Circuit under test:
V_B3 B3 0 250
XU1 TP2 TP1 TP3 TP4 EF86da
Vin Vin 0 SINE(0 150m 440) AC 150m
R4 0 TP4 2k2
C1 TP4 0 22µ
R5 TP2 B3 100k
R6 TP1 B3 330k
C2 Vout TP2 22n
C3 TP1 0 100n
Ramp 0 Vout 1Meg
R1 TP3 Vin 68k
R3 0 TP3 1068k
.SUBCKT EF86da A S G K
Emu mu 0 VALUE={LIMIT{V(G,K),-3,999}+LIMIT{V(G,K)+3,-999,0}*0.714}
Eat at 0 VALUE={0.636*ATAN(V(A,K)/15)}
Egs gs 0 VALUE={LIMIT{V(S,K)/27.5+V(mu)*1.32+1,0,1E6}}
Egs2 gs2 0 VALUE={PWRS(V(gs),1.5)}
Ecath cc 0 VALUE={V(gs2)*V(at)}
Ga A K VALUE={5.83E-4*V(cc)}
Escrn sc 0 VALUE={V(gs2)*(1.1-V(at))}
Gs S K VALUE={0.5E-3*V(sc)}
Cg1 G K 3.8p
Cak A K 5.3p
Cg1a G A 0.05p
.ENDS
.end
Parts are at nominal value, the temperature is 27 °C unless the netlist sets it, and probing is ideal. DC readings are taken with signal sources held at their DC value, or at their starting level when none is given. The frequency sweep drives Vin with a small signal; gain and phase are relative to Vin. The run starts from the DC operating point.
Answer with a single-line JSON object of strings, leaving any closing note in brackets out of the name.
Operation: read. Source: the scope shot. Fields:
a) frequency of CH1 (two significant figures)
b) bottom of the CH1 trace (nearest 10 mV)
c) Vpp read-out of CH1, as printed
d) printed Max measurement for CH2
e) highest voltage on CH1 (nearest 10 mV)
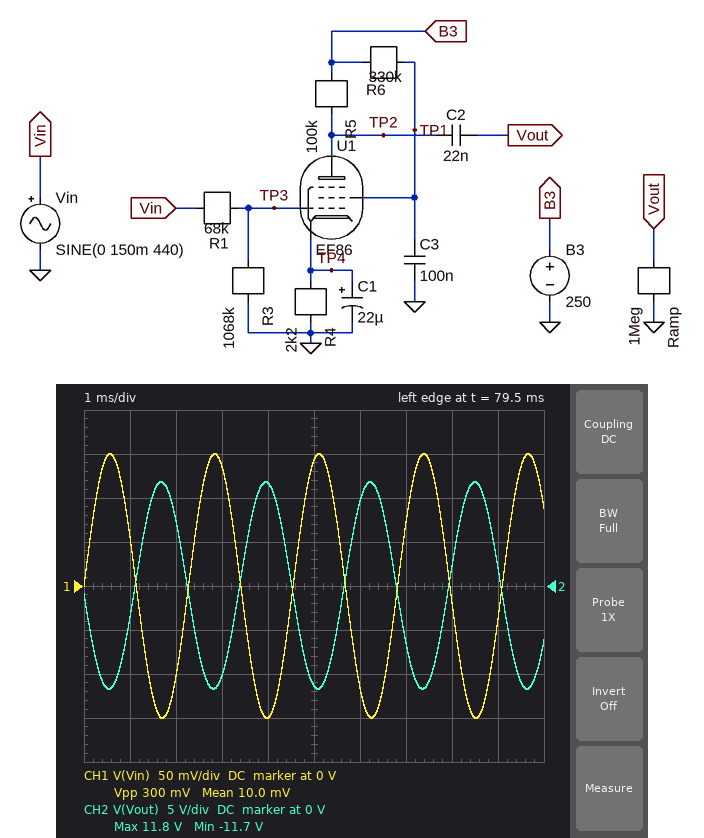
{"frequency of CH1": "440 Hz", "bottom of the CH1 trace": "-150 mV", "Vpp read-out of CH1, as printed": "300 mV", "printed Max measurement for CH2": "11.8 V", "highest voltage on CH1": "150 mV"}
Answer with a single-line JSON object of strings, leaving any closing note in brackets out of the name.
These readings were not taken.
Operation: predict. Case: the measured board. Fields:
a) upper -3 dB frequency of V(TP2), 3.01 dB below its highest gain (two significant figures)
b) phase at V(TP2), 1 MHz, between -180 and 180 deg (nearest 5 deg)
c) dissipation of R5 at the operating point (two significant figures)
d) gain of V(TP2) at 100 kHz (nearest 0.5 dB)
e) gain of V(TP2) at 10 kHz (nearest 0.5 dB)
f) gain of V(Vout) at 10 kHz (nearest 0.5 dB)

{"upper -3 dB frequency of V(TP2), 3.01 dB below its highest gain": "190 kHz", "phase at V(TP2), 1 MHz, between -180 and 180 deg": "60 deg", "dissipation of R5 at the operating point": "210 mW", "gain of V(TP2) at 100 kHz": "37.0 dB", "gain of V(TP2) at 10 kHz": "38.0 dB", "gain of V(Vout) at 10 kHz": "38.0 dB"}
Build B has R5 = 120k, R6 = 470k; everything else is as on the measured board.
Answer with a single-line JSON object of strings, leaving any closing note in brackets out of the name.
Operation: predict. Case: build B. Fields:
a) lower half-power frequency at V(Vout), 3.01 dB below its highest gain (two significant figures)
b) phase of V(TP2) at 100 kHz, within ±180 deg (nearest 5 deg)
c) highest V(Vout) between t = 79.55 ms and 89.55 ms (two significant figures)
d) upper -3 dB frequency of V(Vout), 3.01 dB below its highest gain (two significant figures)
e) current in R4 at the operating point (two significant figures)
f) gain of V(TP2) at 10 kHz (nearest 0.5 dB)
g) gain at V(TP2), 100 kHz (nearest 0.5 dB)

{"lower half-power frequency at V(Vout), 3.01 dB below its highest gain": "31 Hz", "phase of V(TP2) at 100 kHz, within ±180 deg": "145 deg", "highest V(Vout) between t = 79.55 ms and 89.55 ms": "13 V", "upper -3 dB frequency of V(Vout), 3.01 dB below its highest gain": "170 kHz", "current in R4 at the operating point": "1.5 mA", "gain of V(TP2) at 10 kHz": "39.0 dB", "gain at V(TP2), 100 kHz": "37.5 dB"}
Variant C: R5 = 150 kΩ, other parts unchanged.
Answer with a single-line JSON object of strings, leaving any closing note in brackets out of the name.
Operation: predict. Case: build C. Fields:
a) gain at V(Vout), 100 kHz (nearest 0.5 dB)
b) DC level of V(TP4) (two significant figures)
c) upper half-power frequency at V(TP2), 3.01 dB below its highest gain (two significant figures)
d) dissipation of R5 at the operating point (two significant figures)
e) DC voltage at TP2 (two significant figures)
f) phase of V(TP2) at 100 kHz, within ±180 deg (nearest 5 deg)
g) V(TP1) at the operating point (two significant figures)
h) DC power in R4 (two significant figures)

{"gain at V(Vout), 100 kHz": "37.0 dB", "DC level of V(TP4)": "3.4 V", "upper half-power frequency at V(TP2), 3.01 dB below its highest gain": "180 kHz", "dissipation of R5 at the operating point": "230 mW", "DC voltage at TP2": "65 V", "phase of V(TP2) at 100 kHz, within ±180 deg": "145 deg", "V(TP1) at the operating point": "150 V", "DC power in R4": "5.3 mW"}
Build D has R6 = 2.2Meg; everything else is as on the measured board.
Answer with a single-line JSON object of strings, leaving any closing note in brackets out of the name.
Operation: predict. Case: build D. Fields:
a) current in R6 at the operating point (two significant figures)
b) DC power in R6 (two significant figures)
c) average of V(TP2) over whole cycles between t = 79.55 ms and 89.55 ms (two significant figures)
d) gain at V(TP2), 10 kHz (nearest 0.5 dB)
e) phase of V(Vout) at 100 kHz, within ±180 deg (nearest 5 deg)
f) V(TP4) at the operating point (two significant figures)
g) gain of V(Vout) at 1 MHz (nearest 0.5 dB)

{"current in R6 at the operating point": "86 µA", "DC power in R6": "16 mW", "average of V(TP2) over whole cycles between t = 79.55 ms and 89.55 ms": "190 V", "gain at V(TP2), 10 kHz": "39.5 dB", "phase of V(Vout) at 100 kHz, within ±180 deg": "145 deg", "V(TP4) at the operating point": "1.6 V", "gain of V(Vout) at 1 MHz": "22.0 dB"}
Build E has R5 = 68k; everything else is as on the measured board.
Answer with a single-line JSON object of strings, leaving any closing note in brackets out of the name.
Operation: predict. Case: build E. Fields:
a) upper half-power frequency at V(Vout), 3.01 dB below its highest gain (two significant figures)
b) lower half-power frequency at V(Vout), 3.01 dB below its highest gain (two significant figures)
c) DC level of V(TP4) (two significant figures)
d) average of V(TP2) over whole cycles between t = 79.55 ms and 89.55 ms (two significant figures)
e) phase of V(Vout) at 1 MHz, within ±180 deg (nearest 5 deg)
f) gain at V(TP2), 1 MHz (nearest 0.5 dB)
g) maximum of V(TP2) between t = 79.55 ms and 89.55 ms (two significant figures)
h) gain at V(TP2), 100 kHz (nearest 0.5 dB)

{"upper half-power frequency at V(Vout), 3.01 dB below its highest gain": "230 kHz", "lower half-power frequency at V(Vout), 3.01 dB below its highest gain": "28 Hz", "DC level of V(TP4)": "4.0 V", "average of V(TP2) over whole cycles between t = 79.55 ms and 89.55 ms": "140 V", "phase of V(Vout) at 1 MHz, within ±180 deg": "65 deg", "gain at V(TP2), 1 MHz": "21.5 dB", "maximum of V(TP2) between t = 79.55 ms and 89.55 ms": "150 V", "gain at V(TP2), 100 kHz": "35.0 dB"}
